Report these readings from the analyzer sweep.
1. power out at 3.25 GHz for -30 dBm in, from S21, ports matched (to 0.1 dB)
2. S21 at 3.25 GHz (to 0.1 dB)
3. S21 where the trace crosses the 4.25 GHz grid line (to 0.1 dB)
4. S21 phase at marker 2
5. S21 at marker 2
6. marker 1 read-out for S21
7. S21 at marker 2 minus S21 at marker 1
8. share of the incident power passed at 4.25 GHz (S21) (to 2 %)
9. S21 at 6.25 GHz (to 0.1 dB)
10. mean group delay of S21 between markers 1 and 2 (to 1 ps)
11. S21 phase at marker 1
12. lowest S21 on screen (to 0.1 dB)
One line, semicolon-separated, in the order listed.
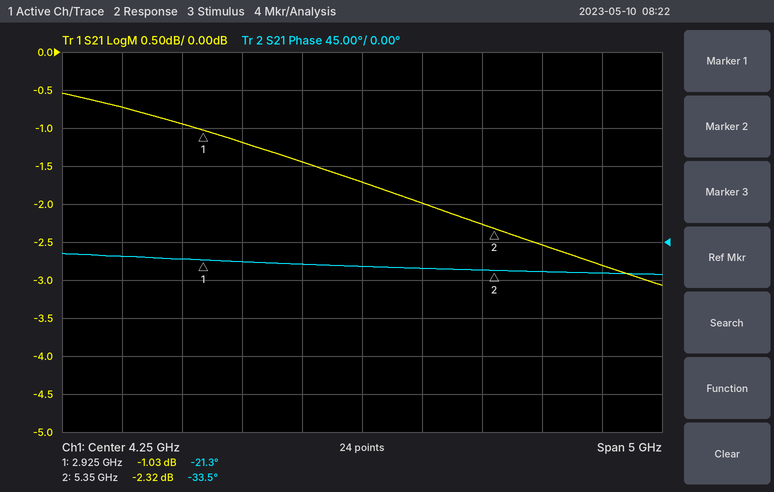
-31.2 dBm; -1.2 dB; -1.7 dB; -33.5°; -2.32 dB; -1.03 dB; -1.29 dB; 68 %; -2.8 dB; 14 ps; -21.3°; -3.1 dB
